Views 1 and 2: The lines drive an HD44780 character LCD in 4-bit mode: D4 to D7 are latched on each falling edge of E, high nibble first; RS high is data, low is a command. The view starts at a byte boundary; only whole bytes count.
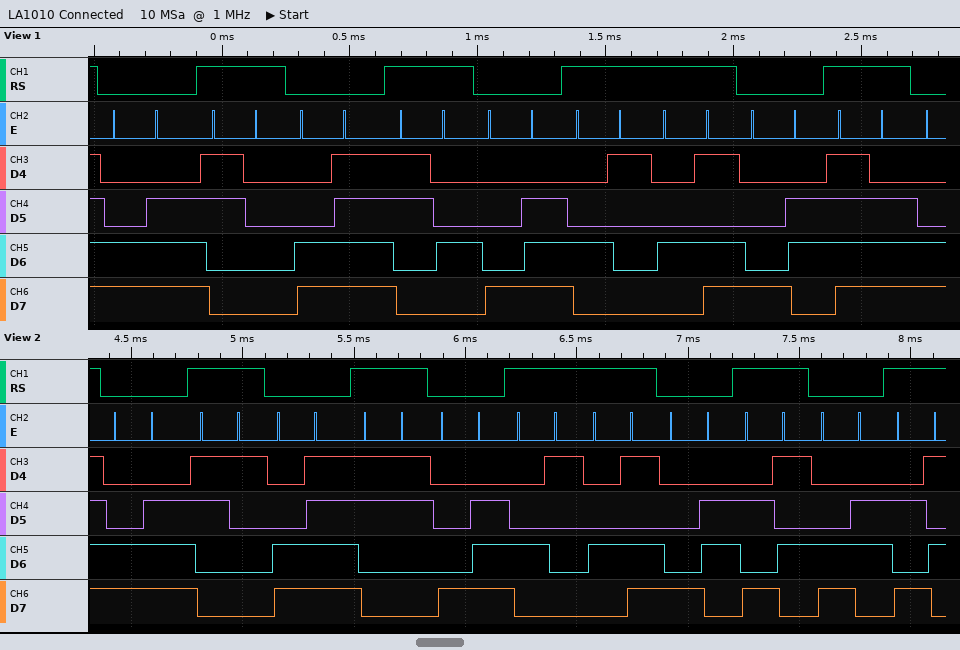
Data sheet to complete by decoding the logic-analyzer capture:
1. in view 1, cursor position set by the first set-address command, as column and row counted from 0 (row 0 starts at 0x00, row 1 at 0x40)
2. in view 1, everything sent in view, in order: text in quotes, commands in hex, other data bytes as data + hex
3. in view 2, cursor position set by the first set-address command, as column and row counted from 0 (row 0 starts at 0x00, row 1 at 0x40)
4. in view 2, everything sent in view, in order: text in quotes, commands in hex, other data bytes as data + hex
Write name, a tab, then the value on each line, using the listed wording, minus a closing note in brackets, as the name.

in view 1, cursor position set by the first set-address command, as column and row counted from 0	column 14, row 1
in view 1, everything sent in view, in order: text in quotes, commands in hex, other data bytes as data + hex	0xCE "0" 0xCF "4" 0x8E "AM" 0x86 data FE
in view 2, cursor position set by the first set-address command, as column and row counted from 0	column 14, row 1
in view 2, everything sent in view, in order: text in quotes, commands in hex, other data bytes as data + hex	0xCE "1" 0xCF "3" 0x8E "AM" 0x86 data A5 0xC6 data A5
